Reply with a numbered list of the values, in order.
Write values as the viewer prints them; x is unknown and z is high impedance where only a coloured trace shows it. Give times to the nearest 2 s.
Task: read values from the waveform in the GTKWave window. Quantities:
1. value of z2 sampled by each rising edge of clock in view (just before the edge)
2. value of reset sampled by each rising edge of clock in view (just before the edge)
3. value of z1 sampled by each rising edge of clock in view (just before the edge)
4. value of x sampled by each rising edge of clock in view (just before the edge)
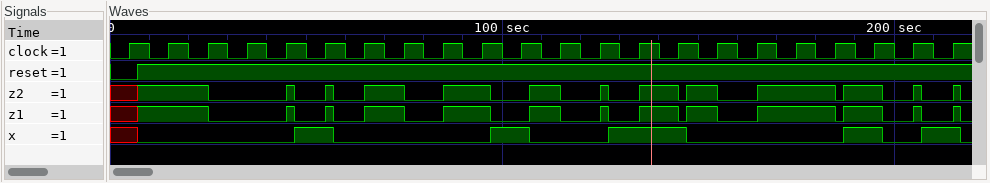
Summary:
1. x 1 1 0 0 0 0 1 0 1 0 1 0 0 1 1 0 1 1 1 0 0
2. 0 1 1 1 1 1 1 1 1 1 1 1 1 1 1 1 1 1 1 1 1 1
3. x 1 1 0 0 0 0 1 0 1 0 1 0 0 1 1 0 1 1 1 0 0
4. x 0 0 0 0 1 0 0 0 0 1 0 0 1 1 0 0 0 0 1 0 1
